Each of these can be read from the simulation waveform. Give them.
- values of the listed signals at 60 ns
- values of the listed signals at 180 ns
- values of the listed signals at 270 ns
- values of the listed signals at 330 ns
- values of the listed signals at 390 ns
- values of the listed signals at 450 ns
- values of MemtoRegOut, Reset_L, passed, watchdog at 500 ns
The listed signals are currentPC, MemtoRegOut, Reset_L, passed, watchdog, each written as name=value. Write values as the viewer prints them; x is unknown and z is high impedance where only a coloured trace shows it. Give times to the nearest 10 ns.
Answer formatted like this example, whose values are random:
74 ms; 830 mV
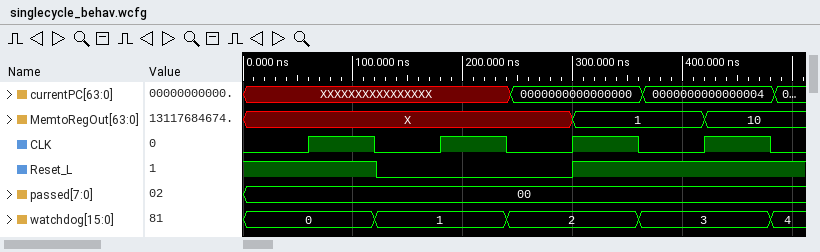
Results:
currentPC=XXXXXXXXXXXXXXXX, MemtoRegOut=X, Reset_L=1, passed=00, watchdog=0; currentPC=XXXXXXXXXXXXXXXX, MemtoRegOut=X, Reset_L=0, passed=00, watchdog=1; currentPC=0000000000000000, MemtoRegOut=X, Reset_L=0, passed=00, watchdog=2; currentPC=0000000000000000, MemtoRegOut=1, Reset_L=1, passed=00, watchdog=2; currentPC=0000000000000004, MemtoRegOut=1, Reset_L=1, passed=00, watchdog=3; currentPC=0000000000000004, MemtoRegOut=10, Reset_L=1, passed=00, watchdog=3; MemtoRegOut=10, Reset_L=1, passed=00, watchdog=4
